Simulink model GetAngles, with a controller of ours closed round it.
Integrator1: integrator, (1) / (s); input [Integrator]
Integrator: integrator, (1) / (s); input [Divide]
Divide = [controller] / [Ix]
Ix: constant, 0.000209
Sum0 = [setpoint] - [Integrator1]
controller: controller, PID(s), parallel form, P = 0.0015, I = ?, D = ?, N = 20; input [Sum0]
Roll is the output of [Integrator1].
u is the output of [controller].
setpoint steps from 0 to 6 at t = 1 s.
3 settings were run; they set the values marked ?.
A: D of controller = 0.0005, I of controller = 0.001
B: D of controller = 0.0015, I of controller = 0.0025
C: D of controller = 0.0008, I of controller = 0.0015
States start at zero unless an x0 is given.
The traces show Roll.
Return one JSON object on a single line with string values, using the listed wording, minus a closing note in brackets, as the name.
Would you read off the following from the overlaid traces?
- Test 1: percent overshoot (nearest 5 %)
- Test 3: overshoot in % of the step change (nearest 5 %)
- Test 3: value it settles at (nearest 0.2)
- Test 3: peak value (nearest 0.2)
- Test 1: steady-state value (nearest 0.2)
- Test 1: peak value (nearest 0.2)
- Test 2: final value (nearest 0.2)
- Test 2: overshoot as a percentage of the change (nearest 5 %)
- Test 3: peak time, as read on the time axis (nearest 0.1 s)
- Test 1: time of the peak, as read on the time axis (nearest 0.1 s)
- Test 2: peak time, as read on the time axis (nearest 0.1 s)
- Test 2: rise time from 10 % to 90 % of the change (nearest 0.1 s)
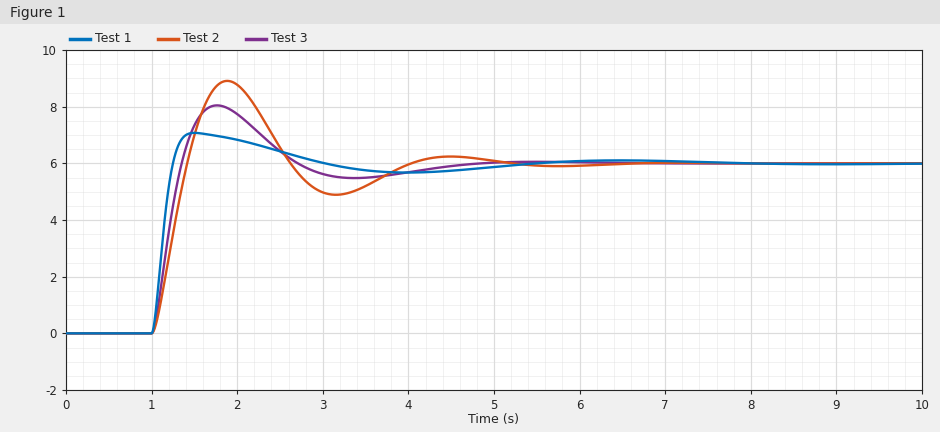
{"Test 1: percent overshoot": "20 %", "Test 3: overshoot in % of the step change": "35 %", "Test 3: value it settles at": "6.0", "Test 3: peak value": "8.0", "Test 1: steady-state value": "6.0", "Test 1: peak value": "7.0", "Test 2: final value": "6.0", "Test 2: overshoot as a percentage of the change": "50 %", "Test 3: peak time, as read on the time axis": "1.8 s", "Test 1: time of the peak, as read on the time axis": "1.5 s", "Test 2: peak time, as read on the time axis": "1.9 s", "Test 2: rise time from 10 % to 90 % of the change": "0.3 s"}
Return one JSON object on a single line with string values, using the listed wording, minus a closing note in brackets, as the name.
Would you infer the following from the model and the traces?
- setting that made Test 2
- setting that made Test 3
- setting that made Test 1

{"setting that made Test 2": "A", "setting that made Test 3": "C", "setting that made Test 1": "B"}
